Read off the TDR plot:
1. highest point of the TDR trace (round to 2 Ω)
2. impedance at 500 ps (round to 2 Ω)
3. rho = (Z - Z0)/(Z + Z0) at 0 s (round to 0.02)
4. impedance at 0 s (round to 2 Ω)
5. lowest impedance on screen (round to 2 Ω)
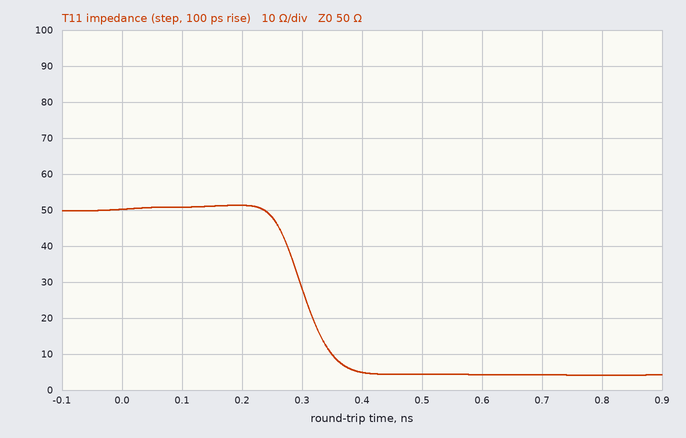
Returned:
52 Ω
4 Ω
0.00
50 Ω
4 Ω
